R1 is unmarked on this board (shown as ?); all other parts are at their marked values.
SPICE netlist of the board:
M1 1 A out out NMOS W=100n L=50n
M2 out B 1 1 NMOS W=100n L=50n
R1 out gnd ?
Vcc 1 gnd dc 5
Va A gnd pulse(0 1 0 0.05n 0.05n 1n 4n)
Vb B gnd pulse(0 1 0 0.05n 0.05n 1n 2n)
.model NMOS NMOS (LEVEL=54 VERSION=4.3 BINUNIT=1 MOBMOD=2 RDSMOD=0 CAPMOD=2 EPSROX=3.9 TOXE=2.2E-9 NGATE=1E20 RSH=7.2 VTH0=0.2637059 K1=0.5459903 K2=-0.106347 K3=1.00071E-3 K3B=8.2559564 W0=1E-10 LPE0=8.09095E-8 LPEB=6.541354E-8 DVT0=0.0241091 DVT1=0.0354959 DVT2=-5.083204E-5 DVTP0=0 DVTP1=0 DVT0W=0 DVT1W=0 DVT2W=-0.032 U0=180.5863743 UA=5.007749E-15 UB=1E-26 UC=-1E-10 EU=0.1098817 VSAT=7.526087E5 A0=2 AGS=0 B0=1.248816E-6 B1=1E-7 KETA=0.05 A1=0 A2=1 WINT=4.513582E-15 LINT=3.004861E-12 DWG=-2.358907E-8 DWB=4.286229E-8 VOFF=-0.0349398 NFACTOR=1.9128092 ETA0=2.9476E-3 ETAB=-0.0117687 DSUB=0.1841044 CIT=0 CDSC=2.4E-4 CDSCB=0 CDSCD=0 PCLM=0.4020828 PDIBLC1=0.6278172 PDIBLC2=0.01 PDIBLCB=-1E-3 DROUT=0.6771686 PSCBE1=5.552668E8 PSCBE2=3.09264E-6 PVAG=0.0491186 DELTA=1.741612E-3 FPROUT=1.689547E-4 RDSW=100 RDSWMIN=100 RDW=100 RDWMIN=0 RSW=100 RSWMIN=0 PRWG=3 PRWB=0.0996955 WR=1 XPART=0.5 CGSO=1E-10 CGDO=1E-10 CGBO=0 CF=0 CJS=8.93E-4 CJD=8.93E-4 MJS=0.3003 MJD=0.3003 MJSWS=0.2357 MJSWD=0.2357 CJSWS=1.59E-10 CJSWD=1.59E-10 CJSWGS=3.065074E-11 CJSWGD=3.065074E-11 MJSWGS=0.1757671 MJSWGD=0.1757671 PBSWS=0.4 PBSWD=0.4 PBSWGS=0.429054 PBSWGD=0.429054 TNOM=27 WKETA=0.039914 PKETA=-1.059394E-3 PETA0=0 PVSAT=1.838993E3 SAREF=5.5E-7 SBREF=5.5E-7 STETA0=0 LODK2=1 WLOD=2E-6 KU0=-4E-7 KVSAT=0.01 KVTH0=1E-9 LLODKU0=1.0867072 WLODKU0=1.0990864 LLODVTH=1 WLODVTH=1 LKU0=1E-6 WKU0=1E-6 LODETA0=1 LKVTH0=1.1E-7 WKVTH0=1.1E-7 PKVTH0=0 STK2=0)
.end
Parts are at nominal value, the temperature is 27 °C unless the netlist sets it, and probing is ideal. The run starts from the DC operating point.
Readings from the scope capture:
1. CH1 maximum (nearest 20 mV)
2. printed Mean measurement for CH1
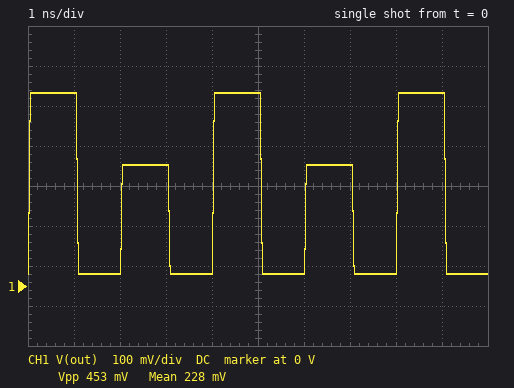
480 mV
228 mV
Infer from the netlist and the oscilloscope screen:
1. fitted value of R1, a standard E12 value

390 Ω
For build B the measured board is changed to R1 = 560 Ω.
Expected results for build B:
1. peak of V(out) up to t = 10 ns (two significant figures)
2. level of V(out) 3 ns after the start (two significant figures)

530 mV
360 mV
